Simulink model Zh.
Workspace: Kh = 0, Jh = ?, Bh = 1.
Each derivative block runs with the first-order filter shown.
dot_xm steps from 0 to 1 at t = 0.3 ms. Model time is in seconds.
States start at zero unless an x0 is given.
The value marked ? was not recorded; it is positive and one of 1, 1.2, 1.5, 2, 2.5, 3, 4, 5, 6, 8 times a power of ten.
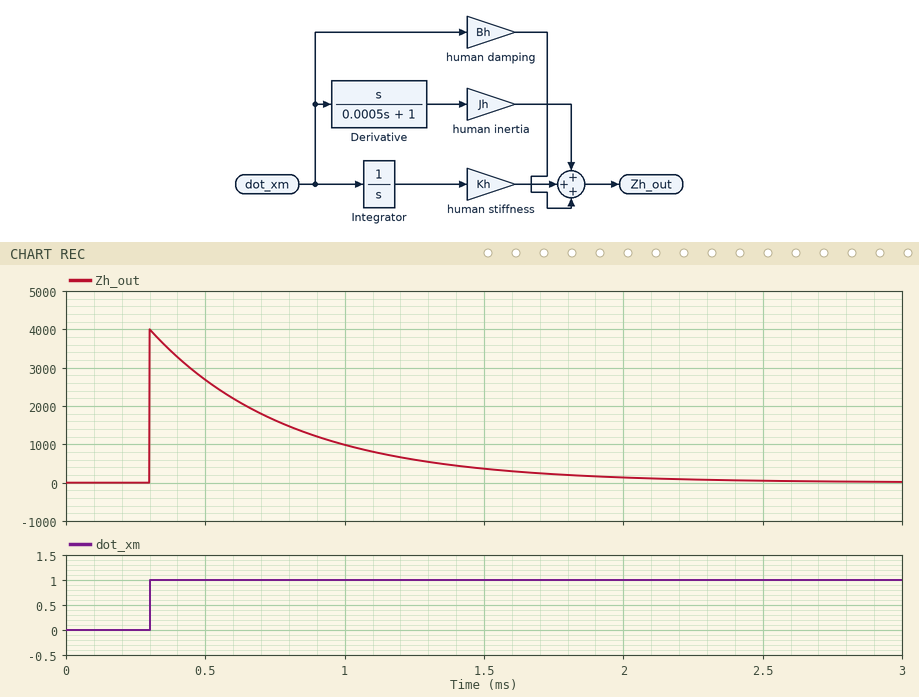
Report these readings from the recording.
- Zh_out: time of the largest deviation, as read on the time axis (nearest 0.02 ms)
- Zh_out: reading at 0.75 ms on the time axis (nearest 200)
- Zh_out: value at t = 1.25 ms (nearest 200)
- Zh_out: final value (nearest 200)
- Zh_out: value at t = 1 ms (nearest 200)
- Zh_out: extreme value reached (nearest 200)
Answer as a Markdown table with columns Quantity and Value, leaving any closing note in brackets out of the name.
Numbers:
| Quantity | Value |
|---|---|
| Zh_out: time of the largest deviation, as read on the time axis | 0.30 ms |
| Zh_out: reading at 0.75 ms on the time axis | 1600 |
| Zh_out: value at t = 1.25 ms | 600 |
| Zh_out: final value | 0 |
| Zh_out: value at t = 1 ms | 1000 |
| Zh_out: extreme value reached | 4000 |
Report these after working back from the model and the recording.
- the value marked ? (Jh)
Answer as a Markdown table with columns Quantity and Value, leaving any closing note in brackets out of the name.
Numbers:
| Quantity | Value |
|---|---|
| the value marked ? | 2 |
